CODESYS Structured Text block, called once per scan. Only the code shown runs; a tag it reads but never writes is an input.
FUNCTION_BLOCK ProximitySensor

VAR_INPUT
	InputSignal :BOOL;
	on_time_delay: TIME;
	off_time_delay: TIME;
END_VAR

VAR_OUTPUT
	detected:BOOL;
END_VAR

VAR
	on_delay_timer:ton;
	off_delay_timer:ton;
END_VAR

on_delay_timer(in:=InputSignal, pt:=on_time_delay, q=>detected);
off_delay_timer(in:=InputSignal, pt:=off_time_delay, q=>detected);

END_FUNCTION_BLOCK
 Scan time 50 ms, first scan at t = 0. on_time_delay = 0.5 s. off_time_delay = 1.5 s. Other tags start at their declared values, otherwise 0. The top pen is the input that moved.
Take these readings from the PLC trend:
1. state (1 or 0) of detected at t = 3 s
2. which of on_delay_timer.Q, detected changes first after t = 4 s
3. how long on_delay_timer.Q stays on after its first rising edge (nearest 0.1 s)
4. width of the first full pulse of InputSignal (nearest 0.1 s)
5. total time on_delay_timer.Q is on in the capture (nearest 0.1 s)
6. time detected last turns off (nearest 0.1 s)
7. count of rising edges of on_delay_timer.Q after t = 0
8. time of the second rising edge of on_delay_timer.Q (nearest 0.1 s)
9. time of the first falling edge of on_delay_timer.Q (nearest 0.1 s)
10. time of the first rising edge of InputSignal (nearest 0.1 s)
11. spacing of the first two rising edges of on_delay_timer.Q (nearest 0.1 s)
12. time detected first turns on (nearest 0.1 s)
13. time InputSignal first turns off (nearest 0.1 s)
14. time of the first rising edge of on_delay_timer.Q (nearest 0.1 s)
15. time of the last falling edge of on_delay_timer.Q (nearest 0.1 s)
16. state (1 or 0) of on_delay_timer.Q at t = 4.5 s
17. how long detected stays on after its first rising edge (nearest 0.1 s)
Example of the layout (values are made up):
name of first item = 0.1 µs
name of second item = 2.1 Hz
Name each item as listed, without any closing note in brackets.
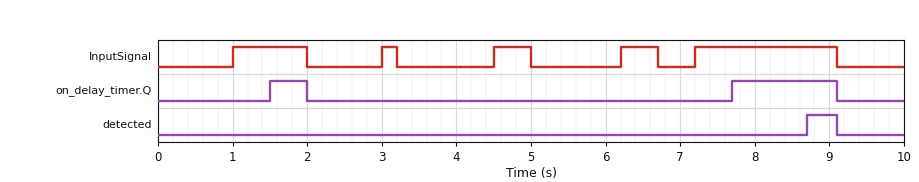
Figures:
state (1 or 0) of detected at t = 3 s = 0
which of on_delay_timer.Q, detected changes first after t = 4 s = on_delay_timer.Q
how long on_delay_timer.Q stays on after its first rising edge = 0.5 s
width of the first full pulse of InputSignal = 1.0 s
total time on_delay_timer.Q is on in the capture = 1.9 s
time detected last turns off = 9.1 s
count of rising edges of on_delay_timer.Q after t = 0 = 2
time of the second rising edge of on_delay_timer.Q = 7.7 s
time of the first falling edge of on_delay_timer.Q = 2.0 s
time of the first rising edge of InputSignal = 1.0 s
spacing of the first two rising edges of on_delay_timer.Q = 6.2 s
time detected first turns on = 8.7 s
time InputSignal first turns off = 2.0 s
time of the first rising edge of on_delay_timer.Q = 1.5 s
time of the last falling edge of on_delay_timer.Q = 9.1 s
state (1 or 0) of on_delay_timer.Q at t = 4.5 s = 0
how long detected stays on after its first rising edge = 0.4 s
